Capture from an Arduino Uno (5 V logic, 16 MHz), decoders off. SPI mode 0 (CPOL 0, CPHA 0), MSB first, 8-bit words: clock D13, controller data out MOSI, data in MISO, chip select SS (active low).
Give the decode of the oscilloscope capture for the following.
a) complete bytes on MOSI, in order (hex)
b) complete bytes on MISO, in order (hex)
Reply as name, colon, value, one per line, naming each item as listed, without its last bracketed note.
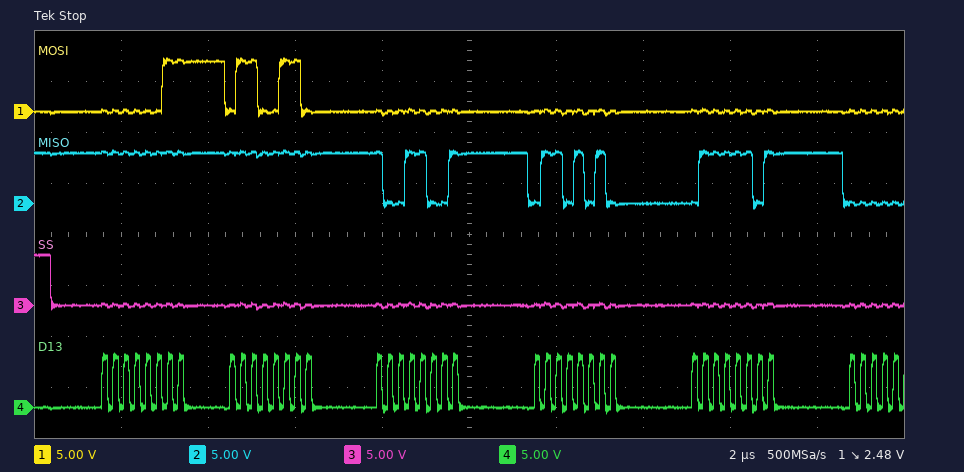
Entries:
complete bytes on MOSI, in order: 03 66 00 00 00
complete bytes on MISO, in order: FF FF 99 6A 7D
